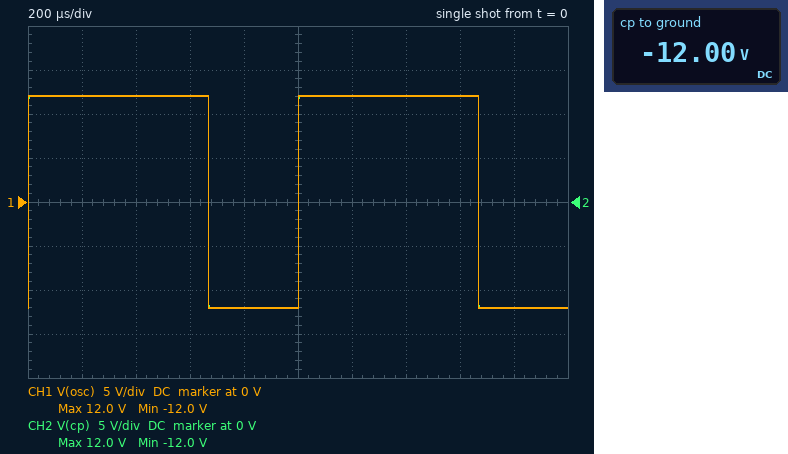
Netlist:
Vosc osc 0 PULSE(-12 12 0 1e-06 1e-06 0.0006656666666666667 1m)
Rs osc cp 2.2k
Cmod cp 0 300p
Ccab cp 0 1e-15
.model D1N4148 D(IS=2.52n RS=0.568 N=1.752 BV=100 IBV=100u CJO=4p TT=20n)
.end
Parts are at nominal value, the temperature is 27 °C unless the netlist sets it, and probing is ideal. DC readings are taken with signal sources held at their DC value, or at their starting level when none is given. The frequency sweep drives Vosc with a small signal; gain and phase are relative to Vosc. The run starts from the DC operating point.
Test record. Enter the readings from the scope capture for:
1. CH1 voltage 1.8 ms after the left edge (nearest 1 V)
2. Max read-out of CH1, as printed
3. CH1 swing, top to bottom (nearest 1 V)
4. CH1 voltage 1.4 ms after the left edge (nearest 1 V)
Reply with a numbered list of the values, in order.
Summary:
1. -12 V
2. 12.0 V
3. 24 V
4. 12 V
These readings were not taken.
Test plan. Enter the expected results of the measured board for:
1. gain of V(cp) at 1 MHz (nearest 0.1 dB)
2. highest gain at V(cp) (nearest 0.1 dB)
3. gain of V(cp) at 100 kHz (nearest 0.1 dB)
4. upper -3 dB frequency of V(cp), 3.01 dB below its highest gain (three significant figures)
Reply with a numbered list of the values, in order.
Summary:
1. -12.6 dB
2. 0 dB
3. -0.7 dB
4. 241 kHz
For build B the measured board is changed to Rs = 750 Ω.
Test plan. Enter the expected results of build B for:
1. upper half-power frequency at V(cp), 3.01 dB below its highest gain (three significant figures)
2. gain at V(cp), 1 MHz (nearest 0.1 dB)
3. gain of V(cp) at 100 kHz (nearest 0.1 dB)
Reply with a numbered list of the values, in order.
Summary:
1. 707 kHz
2. -4.8 dB
3. -0.1 dB
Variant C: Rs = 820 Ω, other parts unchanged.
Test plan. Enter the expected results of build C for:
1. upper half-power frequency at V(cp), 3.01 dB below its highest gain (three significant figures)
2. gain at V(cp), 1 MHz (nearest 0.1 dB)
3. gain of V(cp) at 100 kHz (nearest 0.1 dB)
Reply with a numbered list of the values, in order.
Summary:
1. 647 kHz
2. -5.3 dB
3. -0.1 dB
